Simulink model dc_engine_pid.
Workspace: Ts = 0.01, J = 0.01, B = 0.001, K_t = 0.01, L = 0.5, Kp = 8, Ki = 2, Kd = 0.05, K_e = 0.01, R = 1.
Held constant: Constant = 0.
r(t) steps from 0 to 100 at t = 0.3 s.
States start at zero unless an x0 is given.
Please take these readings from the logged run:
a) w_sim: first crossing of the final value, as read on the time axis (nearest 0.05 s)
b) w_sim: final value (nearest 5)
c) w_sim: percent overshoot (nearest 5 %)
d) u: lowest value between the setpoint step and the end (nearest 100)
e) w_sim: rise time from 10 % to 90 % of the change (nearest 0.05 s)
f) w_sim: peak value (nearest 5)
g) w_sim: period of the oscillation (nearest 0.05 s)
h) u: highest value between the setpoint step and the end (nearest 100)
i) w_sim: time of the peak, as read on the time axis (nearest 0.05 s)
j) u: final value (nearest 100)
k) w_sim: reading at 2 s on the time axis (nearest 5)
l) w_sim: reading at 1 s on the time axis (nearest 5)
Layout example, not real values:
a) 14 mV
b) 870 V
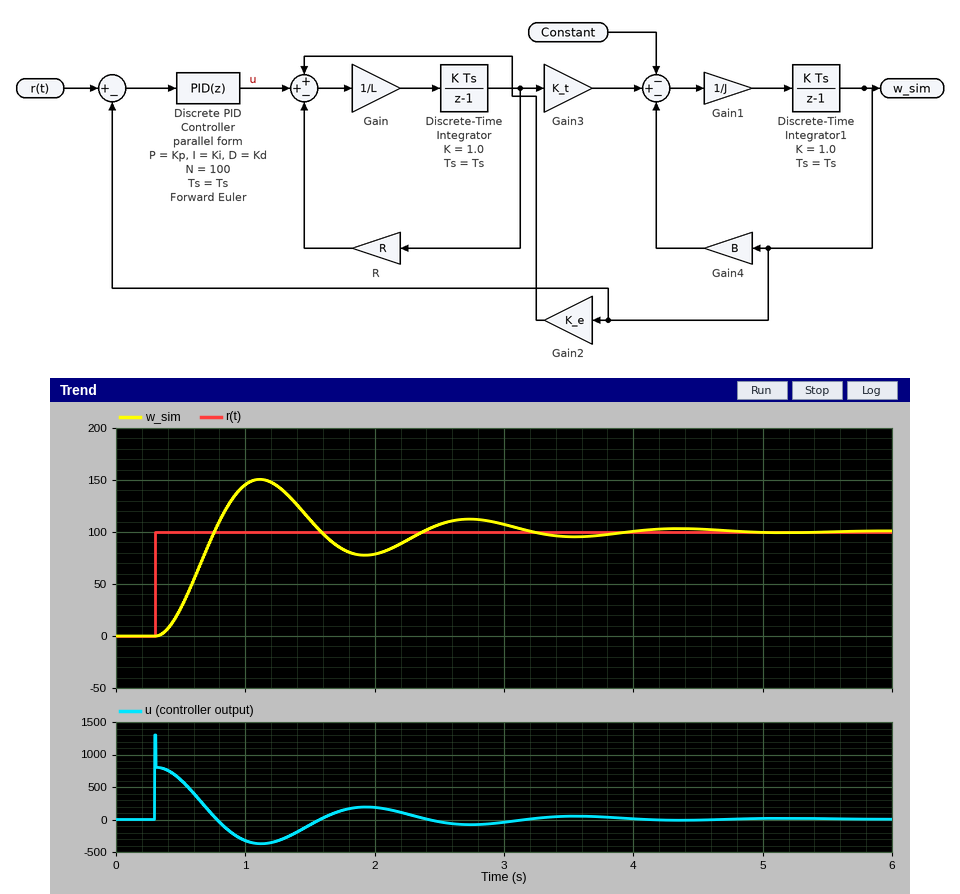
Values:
a) 0.75 s
b) 100
c) 50 %
d) -400
e) 0.30 s
f) 150
g) 1.60 s
h) 1300
i) 1.10 s
j) 0
k) 80
l) 145
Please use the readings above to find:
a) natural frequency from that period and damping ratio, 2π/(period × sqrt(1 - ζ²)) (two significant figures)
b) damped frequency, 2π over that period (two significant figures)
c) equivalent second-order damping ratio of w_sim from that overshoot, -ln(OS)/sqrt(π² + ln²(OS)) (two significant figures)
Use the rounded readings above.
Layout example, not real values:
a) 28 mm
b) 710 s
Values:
a) 4.0 rad/s
b) 3.9 rad/s
c) 0.22
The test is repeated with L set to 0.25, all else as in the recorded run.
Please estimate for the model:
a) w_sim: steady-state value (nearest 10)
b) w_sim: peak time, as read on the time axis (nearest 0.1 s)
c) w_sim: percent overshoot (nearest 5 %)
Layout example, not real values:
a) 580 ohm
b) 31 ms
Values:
a) 100
b) 0.9 s
c) 35 %
